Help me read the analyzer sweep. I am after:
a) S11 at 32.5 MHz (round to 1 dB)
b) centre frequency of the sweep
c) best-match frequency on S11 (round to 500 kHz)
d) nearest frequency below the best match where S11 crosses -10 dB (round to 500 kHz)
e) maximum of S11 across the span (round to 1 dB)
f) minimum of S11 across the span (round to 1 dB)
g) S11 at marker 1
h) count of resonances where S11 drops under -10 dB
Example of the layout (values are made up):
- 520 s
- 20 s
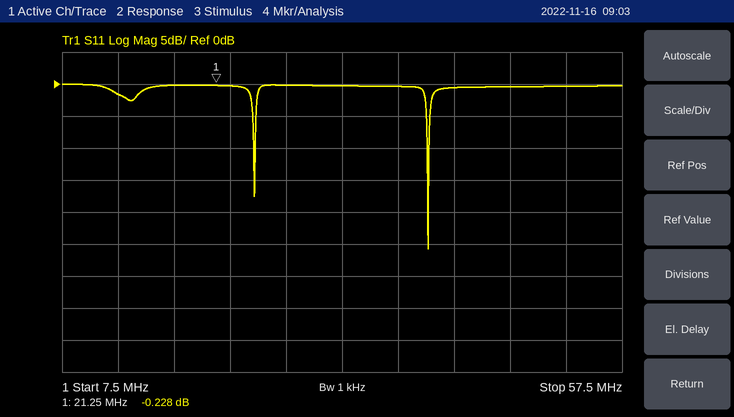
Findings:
- 0 dB
- 32.5 MHz
- 40.0 MHz
- 40.0 MHz
- 0 dB
- -26 dB
- -0.228 dB
- 2
